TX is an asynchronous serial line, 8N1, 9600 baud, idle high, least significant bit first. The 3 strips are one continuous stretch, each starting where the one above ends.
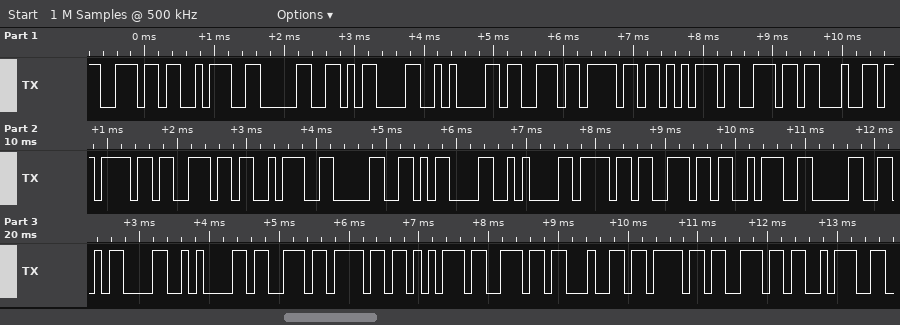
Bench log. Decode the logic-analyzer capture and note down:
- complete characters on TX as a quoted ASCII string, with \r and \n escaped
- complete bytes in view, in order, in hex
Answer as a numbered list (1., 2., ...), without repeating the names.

1. "n:0\r\nsoundon:0\r\non:0\r\nsoundon:"
2. 6E 3A 30 0D 0A 73 6F 75 6E 64 6F 6E 3A 30 0D 0A 6F 6E 3A 30 0D 0A 73 6F 75 6E 64 6F 6E 3A
